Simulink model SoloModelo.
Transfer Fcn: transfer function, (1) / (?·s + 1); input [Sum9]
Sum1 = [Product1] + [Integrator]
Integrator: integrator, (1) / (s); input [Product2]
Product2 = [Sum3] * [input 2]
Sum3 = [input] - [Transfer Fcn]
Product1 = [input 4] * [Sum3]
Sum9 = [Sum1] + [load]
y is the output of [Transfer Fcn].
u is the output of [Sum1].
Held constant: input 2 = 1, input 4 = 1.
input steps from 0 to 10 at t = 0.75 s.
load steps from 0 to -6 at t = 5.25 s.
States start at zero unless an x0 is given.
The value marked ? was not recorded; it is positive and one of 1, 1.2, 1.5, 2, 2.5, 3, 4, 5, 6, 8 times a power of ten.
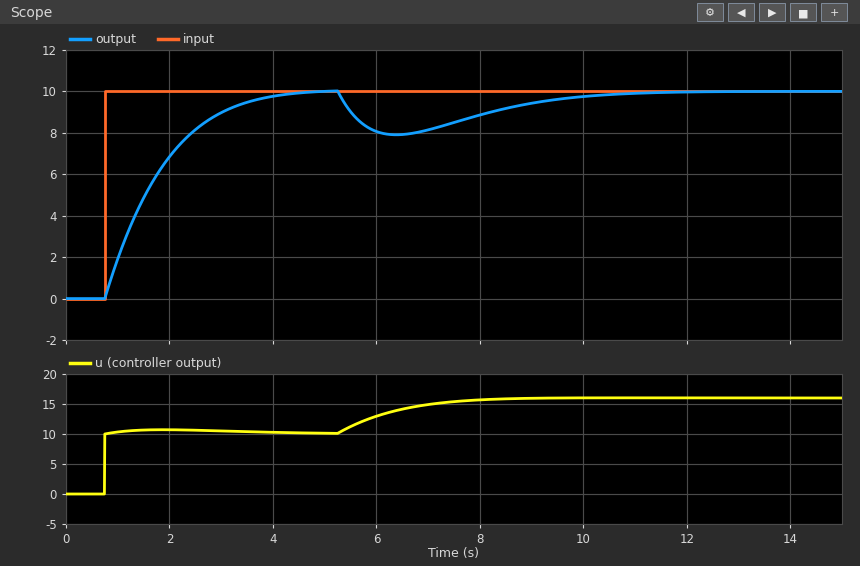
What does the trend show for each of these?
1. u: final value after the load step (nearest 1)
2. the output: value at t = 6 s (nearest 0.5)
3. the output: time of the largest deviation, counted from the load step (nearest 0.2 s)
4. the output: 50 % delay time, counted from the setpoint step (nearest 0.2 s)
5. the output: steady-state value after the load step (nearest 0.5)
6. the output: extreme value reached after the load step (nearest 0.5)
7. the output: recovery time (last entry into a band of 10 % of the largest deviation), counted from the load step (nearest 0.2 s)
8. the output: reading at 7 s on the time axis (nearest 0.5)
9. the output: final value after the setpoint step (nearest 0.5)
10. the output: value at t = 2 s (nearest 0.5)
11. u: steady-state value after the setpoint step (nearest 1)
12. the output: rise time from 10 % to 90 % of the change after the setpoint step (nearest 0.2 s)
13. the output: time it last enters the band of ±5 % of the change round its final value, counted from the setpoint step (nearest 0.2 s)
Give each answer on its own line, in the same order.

16
8.0
1.2 s
0.8 s
10.0
8.0
5.0 s
8.0
10.0
7.0
10
2.2 s
2.8 s
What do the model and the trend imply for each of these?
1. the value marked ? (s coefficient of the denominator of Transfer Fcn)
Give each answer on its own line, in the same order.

1.2
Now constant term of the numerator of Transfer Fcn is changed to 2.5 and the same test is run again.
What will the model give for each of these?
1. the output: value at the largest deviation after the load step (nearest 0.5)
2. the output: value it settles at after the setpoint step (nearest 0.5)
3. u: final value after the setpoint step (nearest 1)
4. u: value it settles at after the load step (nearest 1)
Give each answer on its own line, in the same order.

7.0
10.0
4
10
